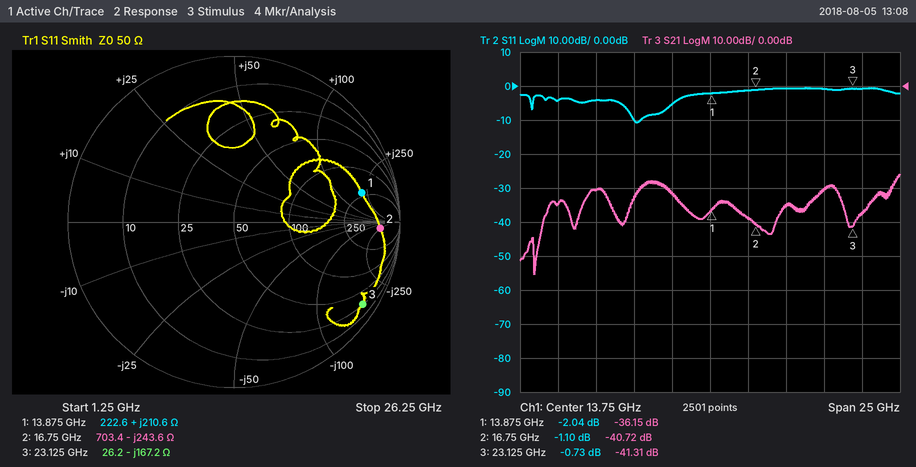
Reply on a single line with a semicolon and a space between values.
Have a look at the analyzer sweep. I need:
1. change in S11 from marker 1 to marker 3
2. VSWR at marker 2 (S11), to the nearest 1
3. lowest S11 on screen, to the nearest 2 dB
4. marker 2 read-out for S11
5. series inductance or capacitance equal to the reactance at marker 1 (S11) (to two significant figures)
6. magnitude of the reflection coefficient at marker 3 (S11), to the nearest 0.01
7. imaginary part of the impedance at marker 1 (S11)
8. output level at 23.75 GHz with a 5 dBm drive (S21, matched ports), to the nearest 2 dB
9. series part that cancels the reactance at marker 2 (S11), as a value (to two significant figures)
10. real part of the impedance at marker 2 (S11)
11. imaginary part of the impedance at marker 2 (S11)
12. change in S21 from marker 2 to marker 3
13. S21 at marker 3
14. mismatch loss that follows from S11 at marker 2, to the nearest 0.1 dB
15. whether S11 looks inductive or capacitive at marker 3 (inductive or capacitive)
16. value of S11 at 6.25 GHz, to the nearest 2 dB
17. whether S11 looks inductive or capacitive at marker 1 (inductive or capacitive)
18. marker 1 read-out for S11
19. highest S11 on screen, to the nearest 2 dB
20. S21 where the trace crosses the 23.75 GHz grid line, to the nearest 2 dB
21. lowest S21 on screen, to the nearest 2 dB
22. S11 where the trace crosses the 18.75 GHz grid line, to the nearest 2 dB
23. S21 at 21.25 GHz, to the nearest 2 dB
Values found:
1.31 dB; 16; -10 dB; -1.10 dB; 2.4 nH; 0.92; +210.6 Ω; -32 dBm; 2.3 nH; 703.4 Ω; -243.6 Ω; -0.59 dB; -41.31 dB; 6.5 dB; capacitive; -4 dB; inductive; -2.04 dB; 0 dB; -38 dB; -56 dB; 0 dB; -30 dB
